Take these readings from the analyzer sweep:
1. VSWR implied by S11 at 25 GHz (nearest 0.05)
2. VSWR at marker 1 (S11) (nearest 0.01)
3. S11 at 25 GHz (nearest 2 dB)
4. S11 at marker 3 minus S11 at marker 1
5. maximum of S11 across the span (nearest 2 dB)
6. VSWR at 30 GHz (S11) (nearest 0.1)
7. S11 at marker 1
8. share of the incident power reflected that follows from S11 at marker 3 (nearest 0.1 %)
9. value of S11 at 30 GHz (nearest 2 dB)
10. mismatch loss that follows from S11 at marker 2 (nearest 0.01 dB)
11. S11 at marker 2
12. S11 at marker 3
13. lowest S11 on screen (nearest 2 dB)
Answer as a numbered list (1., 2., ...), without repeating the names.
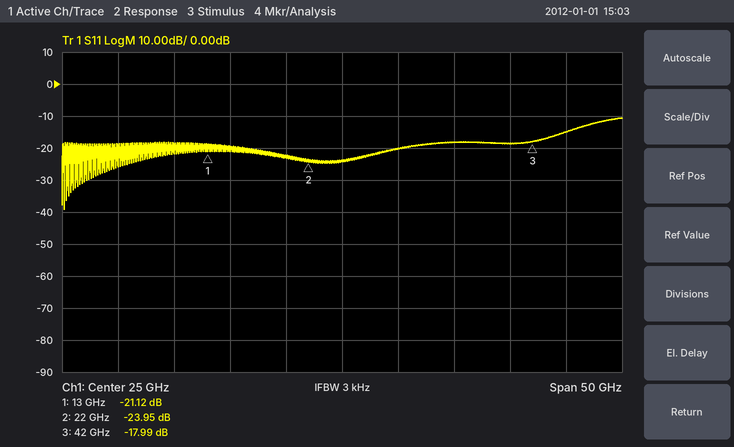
1. 1.15
2. 1.19
3. -24 dB
4. 3.13 dB
5. -10 dB
6. 1.2
7. -21.12 dB
8. 1.6 %
9. -20 dB
10. 0.02 dB
11. -23.95 dB
12. -17.99 dB
13. -40 dB
